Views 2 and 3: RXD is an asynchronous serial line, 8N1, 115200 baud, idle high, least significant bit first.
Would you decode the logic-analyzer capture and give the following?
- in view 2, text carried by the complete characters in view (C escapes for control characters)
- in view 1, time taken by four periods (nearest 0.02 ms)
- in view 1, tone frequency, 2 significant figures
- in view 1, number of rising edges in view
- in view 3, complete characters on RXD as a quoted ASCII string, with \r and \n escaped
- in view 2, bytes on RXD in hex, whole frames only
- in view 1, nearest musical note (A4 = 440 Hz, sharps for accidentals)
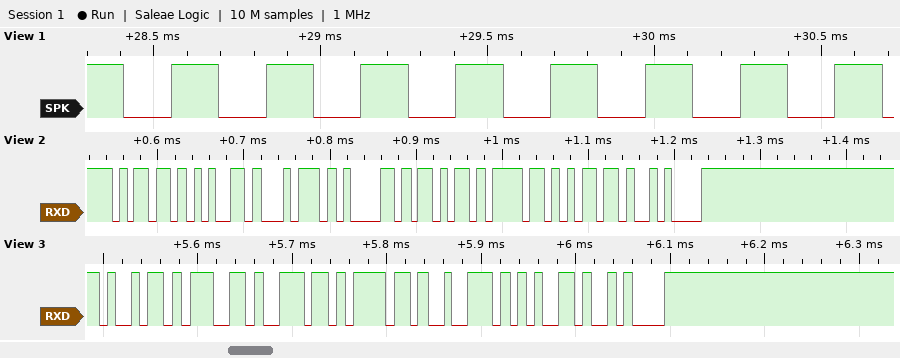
"metakom\n"
1.14 ms
3.5 kHz
8
"ignore\n"
6D 65 74 61 6B 6F 6D 0A
A7
